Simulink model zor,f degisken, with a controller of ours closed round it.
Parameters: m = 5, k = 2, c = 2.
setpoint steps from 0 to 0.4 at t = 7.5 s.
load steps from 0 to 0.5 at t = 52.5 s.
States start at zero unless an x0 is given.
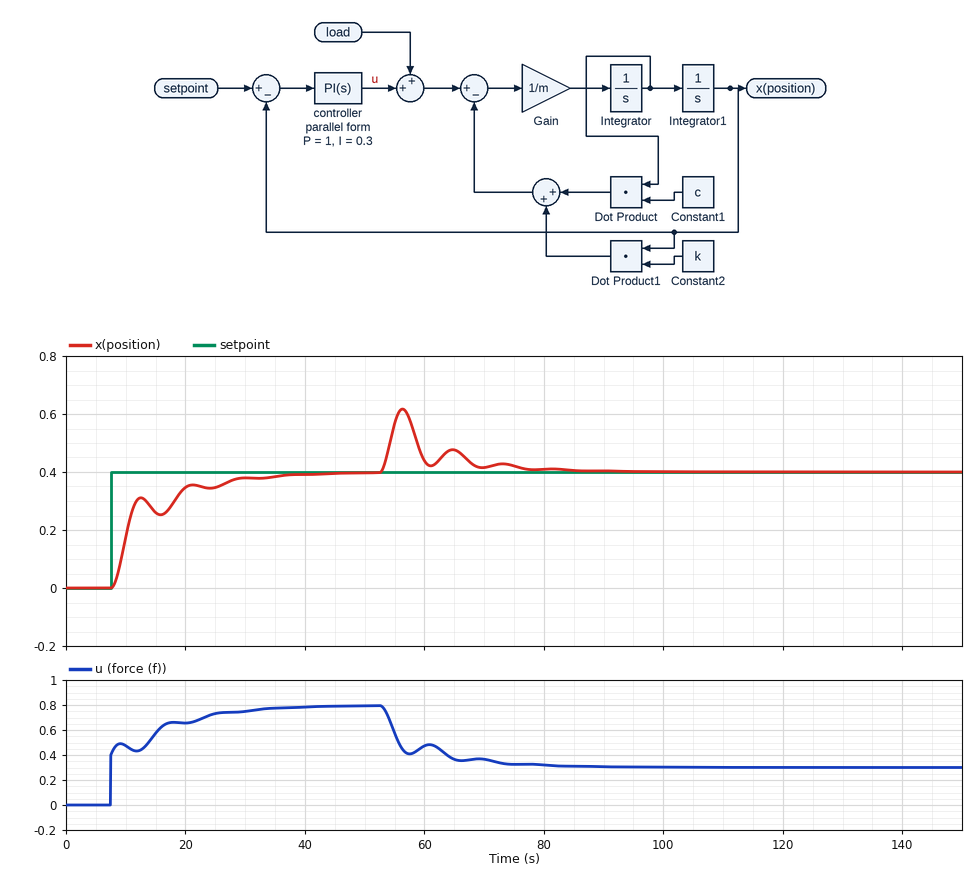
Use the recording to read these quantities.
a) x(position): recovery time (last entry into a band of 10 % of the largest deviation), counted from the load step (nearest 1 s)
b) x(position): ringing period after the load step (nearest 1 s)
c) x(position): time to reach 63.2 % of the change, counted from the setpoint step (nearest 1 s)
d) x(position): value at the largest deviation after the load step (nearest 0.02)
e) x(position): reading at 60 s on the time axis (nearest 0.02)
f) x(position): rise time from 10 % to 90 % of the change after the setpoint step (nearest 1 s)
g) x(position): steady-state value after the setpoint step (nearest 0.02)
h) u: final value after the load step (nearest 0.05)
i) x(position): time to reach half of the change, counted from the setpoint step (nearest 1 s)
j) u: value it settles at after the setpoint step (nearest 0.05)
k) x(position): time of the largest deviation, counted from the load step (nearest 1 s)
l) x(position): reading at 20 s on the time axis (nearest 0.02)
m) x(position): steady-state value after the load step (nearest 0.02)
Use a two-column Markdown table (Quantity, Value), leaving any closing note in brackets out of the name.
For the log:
| Quantity | Value |
|---|---|
| x(position): recovery time (last entry into a band of 10 % of the largest deviation), counted from the load step | 22 s |
| x(position): ringing period after the load step | 8 s |
| x(position): time to reach 63.2 % of the change, counted from the setpoint step | 3 s |
| x(position): value at the largest deviation after the load step | 0.62 |
| x(position): reading at 60 s on the time axis | 0.44 |
| x(position): rise time from 10 % to 90 % of the change after the setpoint step | 18 s |
| x(position): steady-state value after the setpoint step | 0.40 |
| u: final value after the load step | 0.30 |
| x(position): time to reach half of the change, counted from the setpoint step | 3 s |
| u: value it settles at after the setpoint step | 0.80 |
| x(position): time of the largest deviation, counted from the load step | 4 s |
| x(position): reading at 20 s on the time axis | 0.34 |
| x(position): steady-state value after the load step | 0.40 |
